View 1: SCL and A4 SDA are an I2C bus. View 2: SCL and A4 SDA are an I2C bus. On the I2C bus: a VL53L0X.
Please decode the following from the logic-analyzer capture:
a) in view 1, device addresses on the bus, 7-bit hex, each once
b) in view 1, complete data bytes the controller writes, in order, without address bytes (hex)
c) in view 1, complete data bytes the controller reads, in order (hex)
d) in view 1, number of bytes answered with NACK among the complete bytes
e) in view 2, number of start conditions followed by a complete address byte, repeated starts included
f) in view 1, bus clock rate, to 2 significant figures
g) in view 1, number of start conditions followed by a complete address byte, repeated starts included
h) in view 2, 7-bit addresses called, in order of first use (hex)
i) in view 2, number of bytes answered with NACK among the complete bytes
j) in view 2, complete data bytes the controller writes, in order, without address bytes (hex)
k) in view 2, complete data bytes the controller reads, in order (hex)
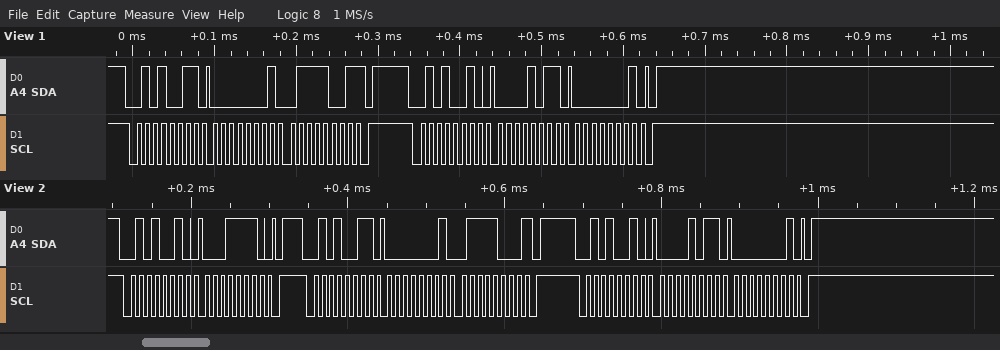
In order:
0x29
0B 01
01 79
1
3
100 kHz
2
0x29
1
1E 0B 01
01 78
